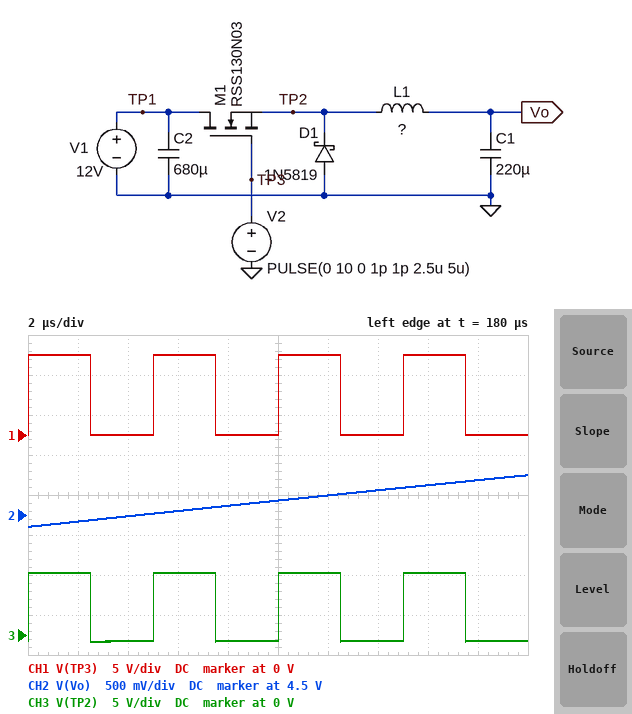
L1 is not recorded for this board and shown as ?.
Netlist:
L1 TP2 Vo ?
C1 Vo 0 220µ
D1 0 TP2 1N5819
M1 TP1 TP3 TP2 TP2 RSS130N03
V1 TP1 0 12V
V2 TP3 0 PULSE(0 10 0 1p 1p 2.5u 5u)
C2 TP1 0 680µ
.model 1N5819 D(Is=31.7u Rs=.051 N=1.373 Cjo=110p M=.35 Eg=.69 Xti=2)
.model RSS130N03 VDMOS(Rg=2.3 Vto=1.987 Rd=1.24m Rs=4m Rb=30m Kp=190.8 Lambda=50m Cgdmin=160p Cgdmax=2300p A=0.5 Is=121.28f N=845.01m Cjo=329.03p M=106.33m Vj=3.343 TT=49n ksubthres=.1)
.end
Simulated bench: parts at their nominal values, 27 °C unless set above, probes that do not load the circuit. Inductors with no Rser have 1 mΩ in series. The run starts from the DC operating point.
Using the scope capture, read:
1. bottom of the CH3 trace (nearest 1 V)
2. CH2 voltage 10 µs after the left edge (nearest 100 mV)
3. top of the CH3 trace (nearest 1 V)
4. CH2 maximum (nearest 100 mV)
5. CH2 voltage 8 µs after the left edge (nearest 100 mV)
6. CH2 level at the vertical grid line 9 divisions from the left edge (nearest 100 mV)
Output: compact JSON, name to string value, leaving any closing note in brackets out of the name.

{"bottom of the CH3 trace": "-1 V", "CH2 voltage 10 µs after the left edge": "4.7 V", "top of the CH3 trace": "8 V", "CH2 maximum": "5.0 V", "CH2 voltage 8 µs after the left edge": "4.6 V", "CH2 level at the vertical grid line 9 divisions from the left edge": "4.9 V"}
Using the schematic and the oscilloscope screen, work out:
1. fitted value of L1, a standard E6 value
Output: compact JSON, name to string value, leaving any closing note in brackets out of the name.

{"fitted value of L1, a standard E6 value": "47 µH"}
